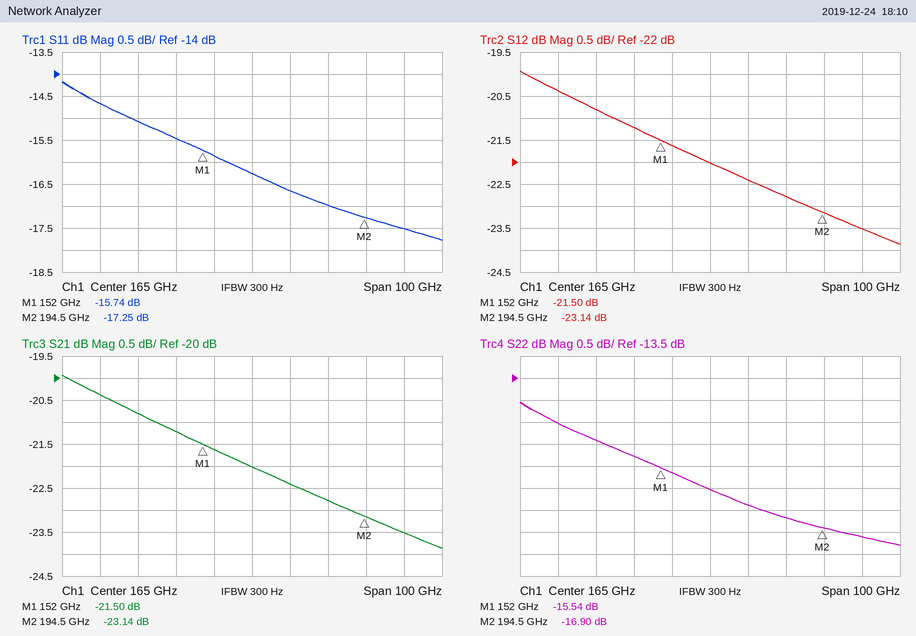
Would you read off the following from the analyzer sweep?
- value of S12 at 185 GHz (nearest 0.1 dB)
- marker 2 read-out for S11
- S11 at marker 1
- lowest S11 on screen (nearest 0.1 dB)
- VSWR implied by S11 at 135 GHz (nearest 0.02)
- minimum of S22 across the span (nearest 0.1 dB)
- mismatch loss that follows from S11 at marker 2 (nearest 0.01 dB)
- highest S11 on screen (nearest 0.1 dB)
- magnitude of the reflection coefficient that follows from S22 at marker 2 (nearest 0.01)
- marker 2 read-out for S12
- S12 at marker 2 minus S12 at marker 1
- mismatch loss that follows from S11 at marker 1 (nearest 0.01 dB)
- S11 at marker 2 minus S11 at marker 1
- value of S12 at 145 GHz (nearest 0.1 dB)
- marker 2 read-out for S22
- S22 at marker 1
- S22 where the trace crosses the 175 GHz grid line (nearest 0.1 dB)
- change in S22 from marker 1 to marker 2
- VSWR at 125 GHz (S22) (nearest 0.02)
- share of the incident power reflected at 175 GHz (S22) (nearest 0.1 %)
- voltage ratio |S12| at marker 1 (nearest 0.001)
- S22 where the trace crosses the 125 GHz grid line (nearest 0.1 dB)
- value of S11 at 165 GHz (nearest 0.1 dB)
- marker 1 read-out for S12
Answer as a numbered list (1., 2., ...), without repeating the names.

1. -22.8 dB
2. -17.25 dB
3. -15.74 dB
4. -17.8 dB
5. 1.42
6. -17.3 dB
7. 0.08 dB
8. -14.2 dB
9. 0.14
10. -23.14 dB
11. -1.64 dB
12. 0.12 dB
13. -1.51 dB
14. -21.2 dB
15. -16.90 dB
16. -15.54 dB
17. -16.4 dB
18. -1.36 dB
19. 1.46
20. 2.3 %
21. 0.084
22. -14.5 dB
23. -16.3 dB
24. -21.50 dB
